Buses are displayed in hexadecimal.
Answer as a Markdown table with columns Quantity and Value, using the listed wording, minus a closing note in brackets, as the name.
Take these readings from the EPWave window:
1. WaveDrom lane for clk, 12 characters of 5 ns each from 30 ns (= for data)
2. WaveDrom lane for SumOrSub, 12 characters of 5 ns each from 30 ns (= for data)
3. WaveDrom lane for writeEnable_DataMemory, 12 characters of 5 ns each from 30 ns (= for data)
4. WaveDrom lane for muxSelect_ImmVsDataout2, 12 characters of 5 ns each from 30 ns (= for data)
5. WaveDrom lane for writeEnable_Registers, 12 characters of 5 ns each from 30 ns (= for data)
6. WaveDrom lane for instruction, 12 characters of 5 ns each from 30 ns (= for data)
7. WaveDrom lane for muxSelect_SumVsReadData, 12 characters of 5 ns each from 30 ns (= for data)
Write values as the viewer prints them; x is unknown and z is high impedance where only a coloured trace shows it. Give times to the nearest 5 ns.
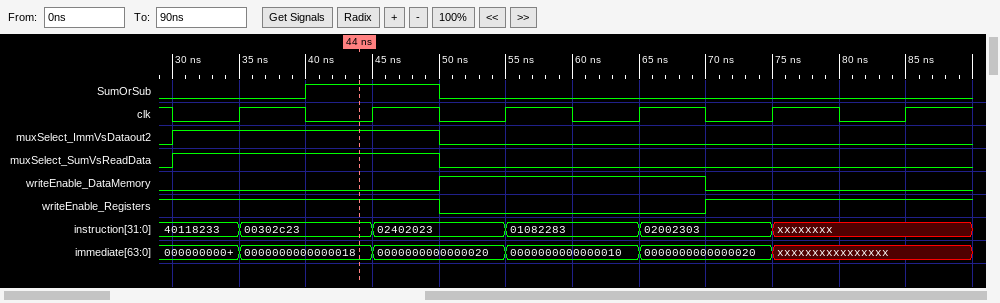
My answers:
| Quantity | Value |
|---|---|
| WaveDrom lane for clk, 12 characters of 5 ns each from 30 ns | {name: 'clk', wave: '010101010101'} |
| WaveDrom lane for SumOrSub, 12 characters of 5 ns each from 30 ns | {name: 'SumOrSub', wave: '0.1.0.......'} |
| WaveDrom lane for writeEnable_DataMemory, 12 characters of 5 ns each from 30 ns | {name: 'writeEnable_DataMemory', wave: '0...1...0...'} |
| WaveDrom lane for muxSelect_ImmVsDataout2, 12 characters of 5 ns each from 30 ns | {name: 'muxSelect_ImmVsDataout2', wave: '1...0.......'} |
| WaveDrom lane for writeEnable_Registers, 12 characters of 5 ns each from 30 ns | {name: 'writeEnable_Registers', wave: '1...0...1...'} |
| WaveDrom lane for instruction, 12 characters of 5 ns each from 30 ns | {name: 'instruction', wave: '==.=.=.=.x..', data: '40118233 00302c23 02402023 01082283 02002303'} |
| WaveDrom lane for muxSelect_SumVsReadData, 12 characters of 5 ns each from 30 ns | {name: 'muxSelect_SumVsReadData', wave: '1...0.......'} |
